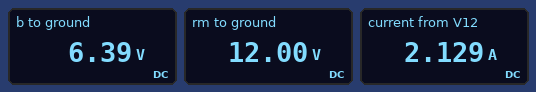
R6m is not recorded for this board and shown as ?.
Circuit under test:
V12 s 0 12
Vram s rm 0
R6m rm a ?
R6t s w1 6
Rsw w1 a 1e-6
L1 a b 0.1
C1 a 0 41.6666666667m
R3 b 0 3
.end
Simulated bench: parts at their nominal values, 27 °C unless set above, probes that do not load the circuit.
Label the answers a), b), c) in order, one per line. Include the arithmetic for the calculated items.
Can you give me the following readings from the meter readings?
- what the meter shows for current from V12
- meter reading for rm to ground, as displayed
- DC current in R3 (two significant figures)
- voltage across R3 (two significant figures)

a) 2.129 A
b) 12.00 V
c) (6.39 V) / 3 Ω = 2.1 A
d) 6.39 V = 6.4 V
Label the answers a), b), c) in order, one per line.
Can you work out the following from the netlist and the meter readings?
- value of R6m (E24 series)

a) 4.7 Ω
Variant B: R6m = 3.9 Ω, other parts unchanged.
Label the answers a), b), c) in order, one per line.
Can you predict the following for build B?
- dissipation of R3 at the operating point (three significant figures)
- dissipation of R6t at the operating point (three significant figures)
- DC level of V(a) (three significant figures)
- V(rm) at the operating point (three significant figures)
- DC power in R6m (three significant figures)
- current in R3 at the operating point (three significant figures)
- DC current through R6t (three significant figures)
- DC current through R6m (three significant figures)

a) 15.0 W
b) 4.66 W
c) 6.71 V
d) 12.0 V
e) 7.17 W
f) 2.24 A
g) 881 mA
h) 1.36 A
